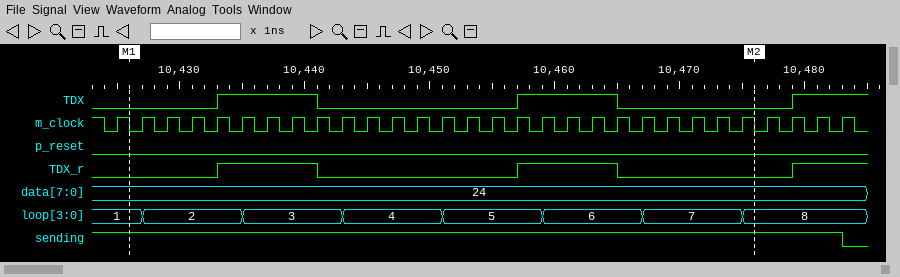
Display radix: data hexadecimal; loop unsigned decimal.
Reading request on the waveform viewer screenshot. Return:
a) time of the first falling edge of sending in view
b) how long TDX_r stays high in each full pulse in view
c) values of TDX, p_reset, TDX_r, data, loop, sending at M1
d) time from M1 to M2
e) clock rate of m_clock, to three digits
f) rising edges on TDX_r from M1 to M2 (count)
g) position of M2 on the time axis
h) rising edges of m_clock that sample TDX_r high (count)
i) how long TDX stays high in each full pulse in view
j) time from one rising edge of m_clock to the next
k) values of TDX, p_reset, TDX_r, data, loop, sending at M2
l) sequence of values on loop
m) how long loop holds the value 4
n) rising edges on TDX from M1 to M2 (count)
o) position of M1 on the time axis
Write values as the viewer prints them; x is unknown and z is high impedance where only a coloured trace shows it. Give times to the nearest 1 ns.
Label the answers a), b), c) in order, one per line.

a) 10483 ns
b) 8 ns, 8 ns
c) TDX=0, p_reset=0, TDX_r=0, data=24, loop=1, sending=1
d) 50 ns
e) 500 MHz
f) 2
g) 10476 ns
h) 10
i) 8 ns, 8 ns
j) 2 ns
k) TDX=0, p_reset=0, TDX_r=0, data=24, loop=8, sending=1
l) 1, 2, 3, 4, 5, 6, 7, 8
m) 8 ns
n) 2
o) 10426 ns
